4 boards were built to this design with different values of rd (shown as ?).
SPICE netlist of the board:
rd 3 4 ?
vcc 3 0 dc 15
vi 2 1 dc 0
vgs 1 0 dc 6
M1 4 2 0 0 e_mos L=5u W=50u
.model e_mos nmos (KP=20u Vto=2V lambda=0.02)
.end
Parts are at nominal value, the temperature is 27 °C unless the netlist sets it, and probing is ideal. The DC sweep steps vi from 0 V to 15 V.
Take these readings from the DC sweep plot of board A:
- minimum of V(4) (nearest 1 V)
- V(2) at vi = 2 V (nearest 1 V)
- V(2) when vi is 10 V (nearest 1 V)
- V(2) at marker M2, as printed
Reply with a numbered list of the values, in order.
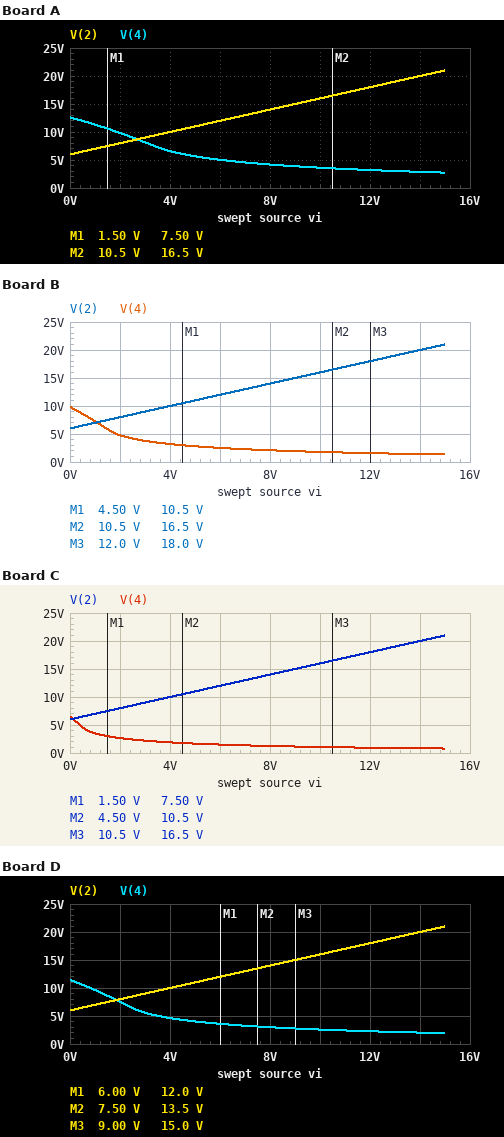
1. 3 V
2. 8 V
3. 16 V
4. 16.5 V
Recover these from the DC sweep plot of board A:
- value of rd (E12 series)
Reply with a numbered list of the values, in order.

1. 1.2 kΩ
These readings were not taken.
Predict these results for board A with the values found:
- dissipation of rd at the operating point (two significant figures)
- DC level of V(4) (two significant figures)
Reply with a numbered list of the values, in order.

1. 4.8 mW
2. 13 V
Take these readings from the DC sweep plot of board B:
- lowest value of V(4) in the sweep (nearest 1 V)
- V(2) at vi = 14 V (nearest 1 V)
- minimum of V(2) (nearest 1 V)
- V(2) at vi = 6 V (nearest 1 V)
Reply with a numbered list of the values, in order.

1. 1 V
2. 20 V
3. 6 V
4. 12 V
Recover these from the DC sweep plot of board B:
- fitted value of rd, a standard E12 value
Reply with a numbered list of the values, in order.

1. 2.7 kΩ
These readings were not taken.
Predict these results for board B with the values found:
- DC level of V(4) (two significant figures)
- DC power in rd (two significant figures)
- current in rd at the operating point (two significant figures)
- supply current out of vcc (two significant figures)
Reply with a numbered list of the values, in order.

1. 9.8 V
2. 9.9 mW
3. 1.9 mA
4. 1.9 mA
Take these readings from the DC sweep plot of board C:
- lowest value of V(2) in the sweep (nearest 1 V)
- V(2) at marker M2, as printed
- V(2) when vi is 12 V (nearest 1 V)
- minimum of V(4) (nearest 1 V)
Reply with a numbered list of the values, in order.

1. 6 V
2. 10.5 V
3. 18 V
4. 1 V
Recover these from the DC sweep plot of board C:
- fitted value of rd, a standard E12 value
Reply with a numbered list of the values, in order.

1. 4.7 kΩ
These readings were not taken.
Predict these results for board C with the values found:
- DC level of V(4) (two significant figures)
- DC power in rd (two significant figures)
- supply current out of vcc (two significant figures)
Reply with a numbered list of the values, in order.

1. 6.5 V
2. 15 mW
3. 1.8 mA
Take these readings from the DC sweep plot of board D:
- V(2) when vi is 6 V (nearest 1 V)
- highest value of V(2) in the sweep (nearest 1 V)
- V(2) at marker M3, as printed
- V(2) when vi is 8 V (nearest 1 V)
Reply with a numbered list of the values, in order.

1. 12 V
2. 21 V
3. 15.0 V
4. 14 V
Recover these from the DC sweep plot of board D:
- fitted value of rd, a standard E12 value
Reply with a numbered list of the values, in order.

1. 1.8 kΩ
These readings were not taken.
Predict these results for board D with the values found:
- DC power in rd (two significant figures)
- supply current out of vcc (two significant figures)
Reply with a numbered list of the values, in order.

1. 7.0 mW
2. 2.0 mA
